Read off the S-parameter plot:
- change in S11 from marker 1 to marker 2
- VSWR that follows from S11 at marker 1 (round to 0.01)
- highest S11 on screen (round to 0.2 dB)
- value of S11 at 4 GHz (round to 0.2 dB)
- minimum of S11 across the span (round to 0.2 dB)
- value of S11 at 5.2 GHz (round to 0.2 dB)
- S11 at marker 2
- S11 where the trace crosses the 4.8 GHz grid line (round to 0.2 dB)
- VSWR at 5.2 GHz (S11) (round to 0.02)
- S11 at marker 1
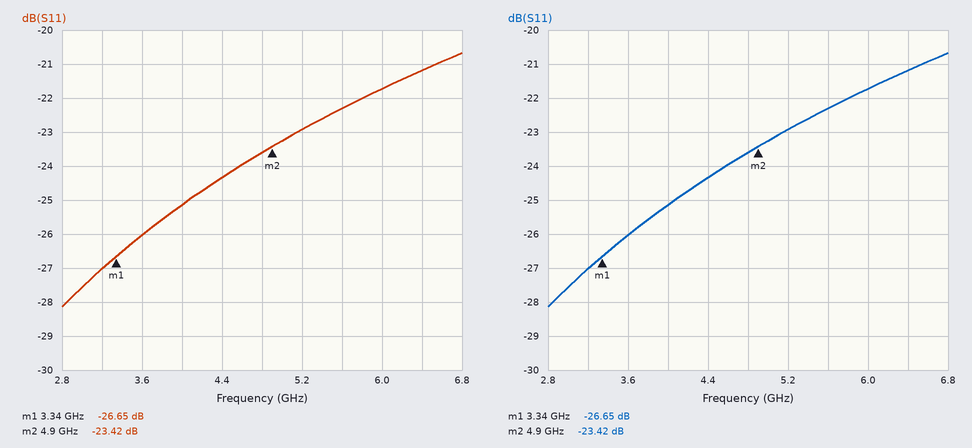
3.23 dB
1.10
-20.6 dB
-25.2 dB
-28.2 dB
-23.0 dB
-23.42 dB
-23.6 dB
1.16
-26.65 dB
